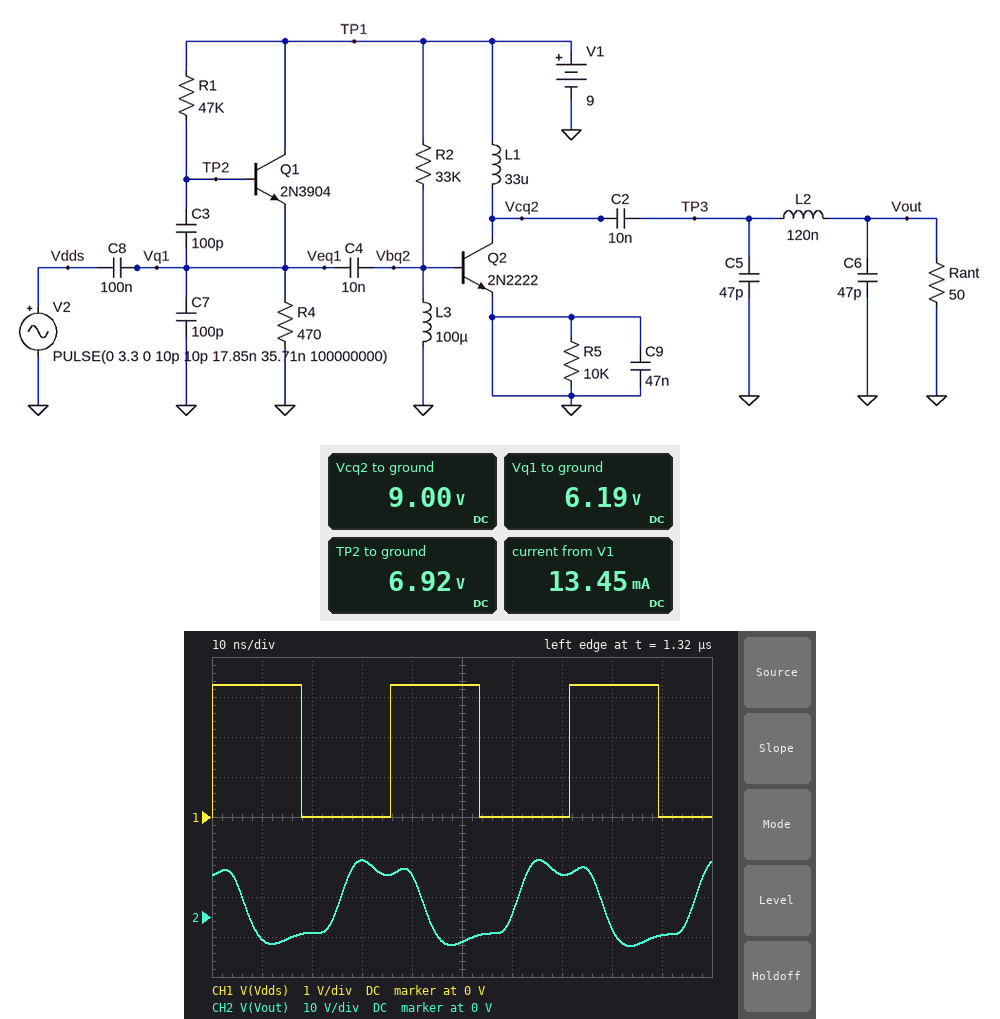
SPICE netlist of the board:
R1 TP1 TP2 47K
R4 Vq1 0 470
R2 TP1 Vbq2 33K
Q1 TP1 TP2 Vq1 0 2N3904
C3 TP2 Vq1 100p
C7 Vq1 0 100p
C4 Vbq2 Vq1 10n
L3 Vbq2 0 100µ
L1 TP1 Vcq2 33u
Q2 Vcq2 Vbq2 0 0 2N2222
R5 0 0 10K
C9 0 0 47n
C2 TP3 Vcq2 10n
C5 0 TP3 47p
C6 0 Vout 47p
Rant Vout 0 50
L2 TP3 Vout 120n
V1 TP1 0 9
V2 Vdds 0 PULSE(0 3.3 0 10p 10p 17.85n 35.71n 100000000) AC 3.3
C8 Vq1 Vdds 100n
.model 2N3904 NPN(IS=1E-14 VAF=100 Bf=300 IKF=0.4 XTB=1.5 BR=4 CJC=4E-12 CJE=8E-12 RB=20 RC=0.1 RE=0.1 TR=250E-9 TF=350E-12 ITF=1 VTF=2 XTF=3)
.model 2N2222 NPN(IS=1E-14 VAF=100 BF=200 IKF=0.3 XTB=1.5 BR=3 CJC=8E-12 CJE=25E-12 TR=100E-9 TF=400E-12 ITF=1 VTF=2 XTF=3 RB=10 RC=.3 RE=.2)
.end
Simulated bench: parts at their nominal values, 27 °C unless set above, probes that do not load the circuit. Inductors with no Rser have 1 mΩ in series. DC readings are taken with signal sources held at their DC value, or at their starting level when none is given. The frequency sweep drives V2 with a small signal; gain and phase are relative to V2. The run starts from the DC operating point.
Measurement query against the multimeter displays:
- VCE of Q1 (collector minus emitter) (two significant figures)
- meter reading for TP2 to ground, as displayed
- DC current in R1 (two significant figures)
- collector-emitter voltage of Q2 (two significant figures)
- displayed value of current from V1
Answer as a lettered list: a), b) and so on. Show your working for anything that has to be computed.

a) 9 V - 6.19 V = 2.8 V
b) 6.92 V
c) (9 V - 6.92 V) / 47 kΩ = 44 µA
d) 9 V = 9.0 V
e) 13.45 mA
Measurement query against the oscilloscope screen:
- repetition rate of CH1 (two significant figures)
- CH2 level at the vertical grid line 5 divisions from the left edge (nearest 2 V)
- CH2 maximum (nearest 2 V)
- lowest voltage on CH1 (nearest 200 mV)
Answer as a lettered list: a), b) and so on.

a) 28 MHz
b) -6 V
c) 14 V
d) 0 V
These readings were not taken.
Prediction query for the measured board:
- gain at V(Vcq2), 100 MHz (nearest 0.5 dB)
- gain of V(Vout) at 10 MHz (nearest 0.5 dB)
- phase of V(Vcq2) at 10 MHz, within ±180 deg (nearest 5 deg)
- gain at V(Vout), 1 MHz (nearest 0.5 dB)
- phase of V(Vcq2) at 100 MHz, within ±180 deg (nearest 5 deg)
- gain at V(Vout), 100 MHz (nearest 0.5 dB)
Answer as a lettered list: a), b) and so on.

a) -17.0 dB
b) -39.5 dB
c) 80 deg
d) -58.5 dB
e) 10 deg
f) -23.0 dB
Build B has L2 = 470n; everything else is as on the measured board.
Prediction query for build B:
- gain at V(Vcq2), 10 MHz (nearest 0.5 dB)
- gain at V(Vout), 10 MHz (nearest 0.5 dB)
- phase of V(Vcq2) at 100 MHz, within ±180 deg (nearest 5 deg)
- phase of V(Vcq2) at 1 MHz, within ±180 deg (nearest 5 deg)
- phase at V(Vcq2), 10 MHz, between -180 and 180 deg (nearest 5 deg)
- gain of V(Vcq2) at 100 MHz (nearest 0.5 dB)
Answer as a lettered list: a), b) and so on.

a) -38.5 dB
b) -39.0 dB
c) -10 deg
d) 90 deg
e) 105 deg
f) -22.5 dB
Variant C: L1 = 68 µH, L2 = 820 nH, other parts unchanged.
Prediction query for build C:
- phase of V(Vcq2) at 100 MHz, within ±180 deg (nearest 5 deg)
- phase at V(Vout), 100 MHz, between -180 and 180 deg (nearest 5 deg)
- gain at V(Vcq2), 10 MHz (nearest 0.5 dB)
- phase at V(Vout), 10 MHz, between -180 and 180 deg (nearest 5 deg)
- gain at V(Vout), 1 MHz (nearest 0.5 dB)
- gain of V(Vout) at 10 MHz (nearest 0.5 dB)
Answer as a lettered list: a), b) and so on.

a) -10 deg
b) -155 deg
c) -36.0 dB
d) 70 deg
e) -59.0 dB
f) -38.5 dB
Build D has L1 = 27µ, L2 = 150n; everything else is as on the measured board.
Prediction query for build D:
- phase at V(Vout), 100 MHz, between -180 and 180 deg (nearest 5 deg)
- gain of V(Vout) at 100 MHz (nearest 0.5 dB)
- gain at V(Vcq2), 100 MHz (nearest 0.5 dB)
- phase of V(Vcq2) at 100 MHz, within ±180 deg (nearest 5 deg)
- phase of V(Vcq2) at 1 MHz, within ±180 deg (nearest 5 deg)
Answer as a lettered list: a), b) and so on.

a) -135 deg
b) -27.0 dB
c) -19.0 dB
d) 0 deg
e) 90 deg
